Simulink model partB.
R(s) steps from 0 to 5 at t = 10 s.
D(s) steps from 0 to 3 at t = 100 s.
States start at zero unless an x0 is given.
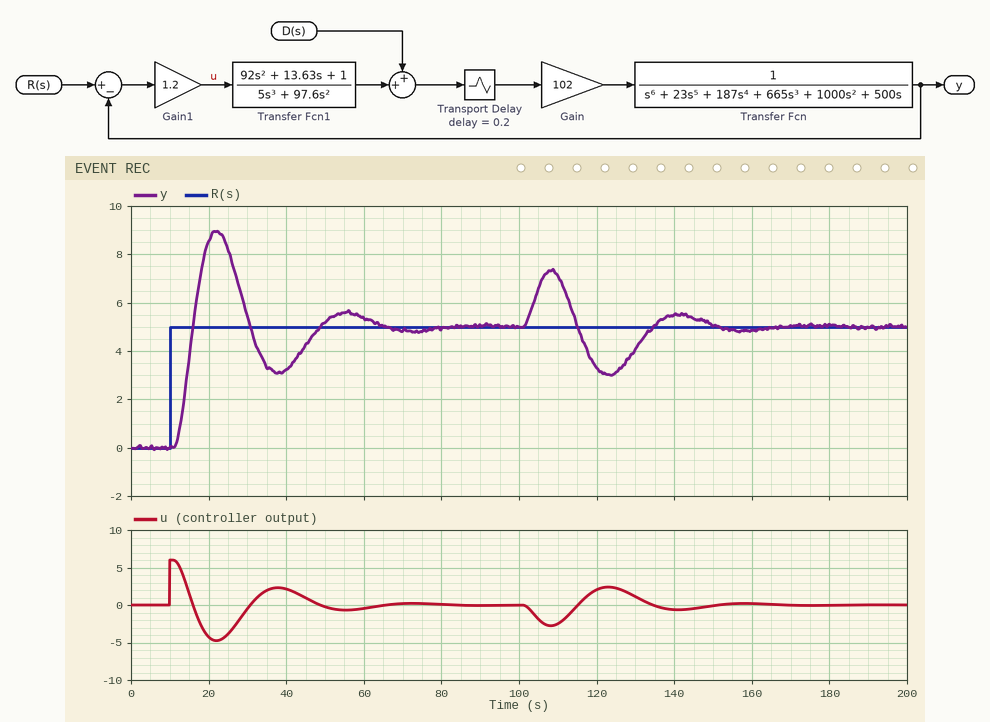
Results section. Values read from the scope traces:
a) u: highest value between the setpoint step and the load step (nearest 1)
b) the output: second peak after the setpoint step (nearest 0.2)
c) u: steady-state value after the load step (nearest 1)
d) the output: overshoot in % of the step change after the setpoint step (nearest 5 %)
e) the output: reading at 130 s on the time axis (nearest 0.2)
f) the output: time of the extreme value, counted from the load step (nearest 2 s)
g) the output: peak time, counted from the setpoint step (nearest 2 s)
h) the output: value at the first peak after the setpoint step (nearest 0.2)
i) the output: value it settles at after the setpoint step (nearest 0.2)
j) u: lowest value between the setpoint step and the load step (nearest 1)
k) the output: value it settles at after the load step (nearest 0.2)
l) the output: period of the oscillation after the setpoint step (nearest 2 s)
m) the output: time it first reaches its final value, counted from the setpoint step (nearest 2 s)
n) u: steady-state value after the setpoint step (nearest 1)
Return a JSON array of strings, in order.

["6", "5.6", "0", "80 %", "4.0", "8 s", "12 s", "9.0", "5.0", "-5", "5.0", "34 s", "6 s", "0"]
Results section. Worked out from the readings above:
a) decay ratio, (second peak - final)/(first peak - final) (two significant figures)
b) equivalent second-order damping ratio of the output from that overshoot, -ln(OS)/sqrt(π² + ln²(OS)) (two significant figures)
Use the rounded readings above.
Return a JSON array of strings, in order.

["0.15", "0.071"]
